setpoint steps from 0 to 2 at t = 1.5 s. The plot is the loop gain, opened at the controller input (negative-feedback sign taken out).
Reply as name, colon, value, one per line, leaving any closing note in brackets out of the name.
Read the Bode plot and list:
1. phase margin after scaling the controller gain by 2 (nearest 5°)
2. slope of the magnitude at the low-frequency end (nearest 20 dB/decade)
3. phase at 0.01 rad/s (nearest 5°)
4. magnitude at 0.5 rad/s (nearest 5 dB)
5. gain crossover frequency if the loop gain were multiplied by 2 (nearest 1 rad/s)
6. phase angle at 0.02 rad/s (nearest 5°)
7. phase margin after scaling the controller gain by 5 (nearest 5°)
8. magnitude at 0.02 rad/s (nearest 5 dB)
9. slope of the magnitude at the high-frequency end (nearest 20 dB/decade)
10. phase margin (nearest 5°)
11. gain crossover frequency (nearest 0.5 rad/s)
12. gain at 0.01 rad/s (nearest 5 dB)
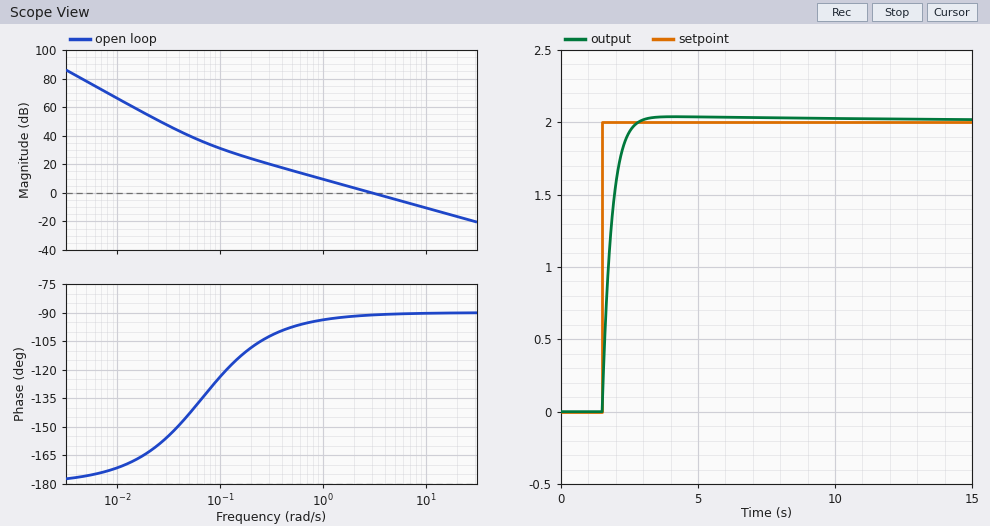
phase margin after scaling the controller gain by 2: 90°
slope of the magnitude at the low-frequency end: -40 dB/decade
phase at 0.01 rad/s: -170°
magnitude at 0.5 rad/s: 15 dB
gain crossover frequency if the loop gain were multiplied by 2: 6 rad/s
phase angle at 0.02 rad/s: -165°
phase margin after scaling the controller gain by 5: 90°
magnitude at 0.02 rad/s: 55 dB
slope of the magnitude at the high-frequency end: -20 dB/decade
phase margin: 90°
gain crossover frequency: 3.0 rad/s
gain at 0.01 rad/s: 65 dB
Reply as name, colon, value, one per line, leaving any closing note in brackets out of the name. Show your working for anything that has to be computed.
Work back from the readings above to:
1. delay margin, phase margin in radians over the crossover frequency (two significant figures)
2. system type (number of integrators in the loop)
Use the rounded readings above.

delay margin, phase margin in radians over the crossover frequency: 90 × π / 180 / 3 = 0.52 s
system type: 2
